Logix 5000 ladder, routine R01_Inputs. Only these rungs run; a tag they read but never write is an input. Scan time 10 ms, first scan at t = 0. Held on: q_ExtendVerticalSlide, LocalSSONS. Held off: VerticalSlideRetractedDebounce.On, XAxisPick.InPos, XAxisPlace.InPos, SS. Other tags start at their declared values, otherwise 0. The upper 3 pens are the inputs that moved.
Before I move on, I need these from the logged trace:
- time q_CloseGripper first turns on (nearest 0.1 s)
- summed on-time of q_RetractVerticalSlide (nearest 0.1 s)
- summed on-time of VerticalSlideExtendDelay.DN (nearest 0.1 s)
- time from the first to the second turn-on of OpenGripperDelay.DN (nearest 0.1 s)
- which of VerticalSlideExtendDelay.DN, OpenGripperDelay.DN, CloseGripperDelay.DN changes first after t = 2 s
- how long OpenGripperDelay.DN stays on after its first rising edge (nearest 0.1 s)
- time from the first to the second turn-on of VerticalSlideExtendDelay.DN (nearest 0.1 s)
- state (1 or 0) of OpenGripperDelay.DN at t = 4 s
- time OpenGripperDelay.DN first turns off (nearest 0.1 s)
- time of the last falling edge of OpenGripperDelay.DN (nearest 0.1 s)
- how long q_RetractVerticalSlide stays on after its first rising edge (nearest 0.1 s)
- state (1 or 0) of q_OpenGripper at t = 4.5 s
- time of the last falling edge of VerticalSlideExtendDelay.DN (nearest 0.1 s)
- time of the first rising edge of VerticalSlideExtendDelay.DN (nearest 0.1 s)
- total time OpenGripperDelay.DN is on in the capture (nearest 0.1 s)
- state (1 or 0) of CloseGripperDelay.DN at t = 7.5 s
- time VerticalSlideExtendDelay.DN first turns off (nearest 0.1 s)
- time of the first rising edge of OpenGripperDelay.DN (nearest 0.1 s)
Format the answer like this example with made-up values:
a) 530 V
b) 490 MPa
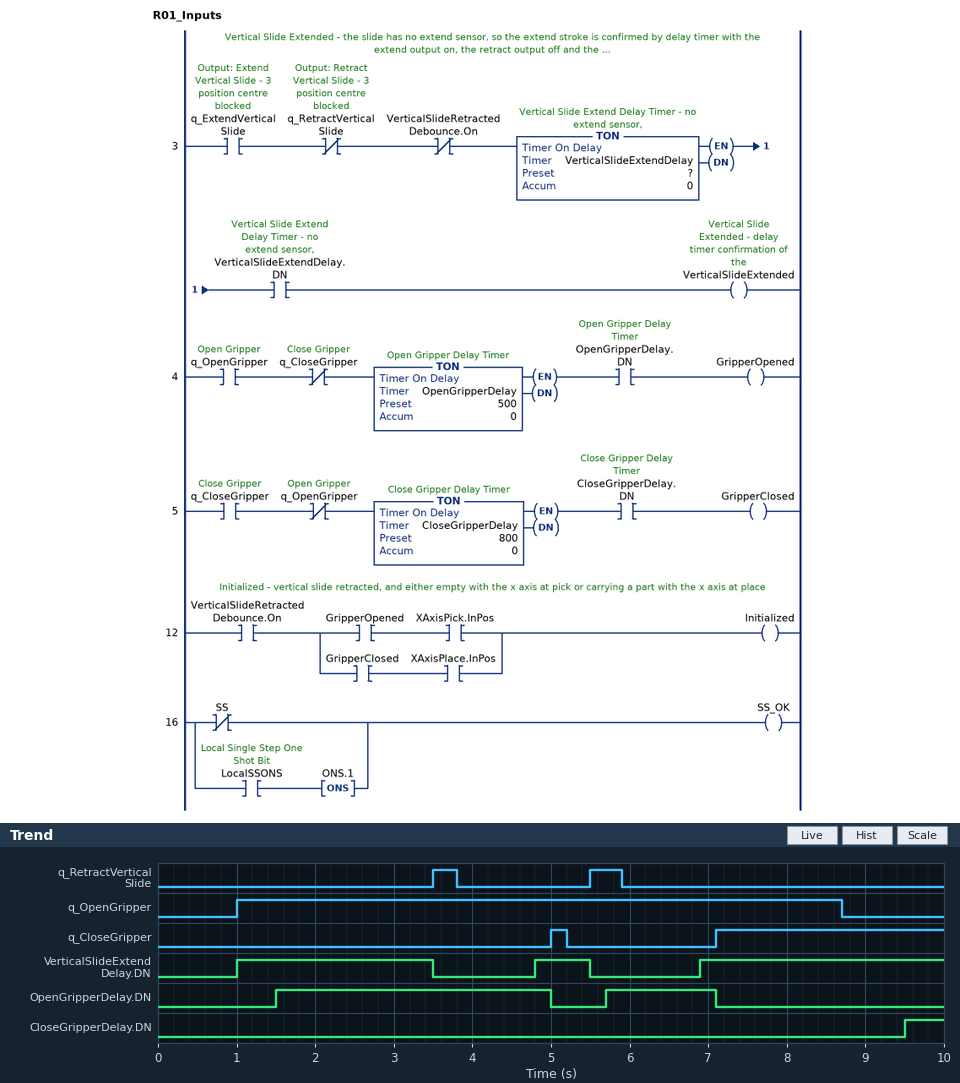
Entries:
a) 5.0 s
b) 0.7 s
c) 6.3 s
d) 4.2 s
e) VerticalSlideExtendDelay.DN
f) 3.5 s
g) 3.8 s
h) 1
i) 5.0 s
j) 7.1 s
k) 0.3 s
l) 1
m) 5.5 s
n) 1.0 s
o) 4.9 s
p) 0
q) 3.5 s
r) 1.5 s
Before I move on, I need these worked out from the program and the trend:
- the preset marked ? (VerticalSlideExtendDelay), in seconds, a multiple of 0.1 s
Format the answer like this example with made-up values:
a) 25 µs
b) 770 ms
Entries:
a) 1.0 s
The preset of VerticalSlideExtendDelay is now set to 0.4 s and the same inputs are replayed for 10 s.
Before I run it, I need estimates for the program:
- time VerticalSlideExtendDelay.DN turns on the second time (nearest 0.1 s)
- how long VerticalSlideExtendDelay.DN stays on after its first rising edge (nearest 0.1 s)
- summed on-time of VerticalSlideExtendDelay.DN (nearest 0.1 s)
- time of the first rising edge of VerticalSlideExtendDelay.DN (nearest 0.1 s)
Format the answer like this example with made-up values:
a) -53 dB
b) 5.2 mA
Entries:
a) 4.2 s
b) 3.1 s
c) 8.1 s
d) 0.4 s
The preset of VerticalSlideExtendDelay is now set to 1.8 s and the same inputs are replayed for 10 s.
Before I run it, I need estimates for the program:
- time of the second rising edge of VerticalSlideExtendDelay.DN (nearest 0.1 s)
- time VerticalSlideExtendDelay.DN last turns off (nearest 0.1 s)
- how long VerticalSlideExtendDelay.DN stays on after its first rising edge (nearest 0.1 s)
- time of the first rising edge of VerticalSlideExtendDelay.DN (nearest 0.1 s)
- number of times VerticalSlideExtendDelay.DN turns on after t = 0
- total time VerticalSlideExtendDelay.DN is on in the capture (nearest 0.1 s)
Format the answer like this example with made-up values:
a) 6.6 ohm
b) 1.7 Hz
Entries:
a) 7.7 s
b) 3.5 s
c) 1.7 s
d) 1.8 s
e) 2
f) 4.0 s
